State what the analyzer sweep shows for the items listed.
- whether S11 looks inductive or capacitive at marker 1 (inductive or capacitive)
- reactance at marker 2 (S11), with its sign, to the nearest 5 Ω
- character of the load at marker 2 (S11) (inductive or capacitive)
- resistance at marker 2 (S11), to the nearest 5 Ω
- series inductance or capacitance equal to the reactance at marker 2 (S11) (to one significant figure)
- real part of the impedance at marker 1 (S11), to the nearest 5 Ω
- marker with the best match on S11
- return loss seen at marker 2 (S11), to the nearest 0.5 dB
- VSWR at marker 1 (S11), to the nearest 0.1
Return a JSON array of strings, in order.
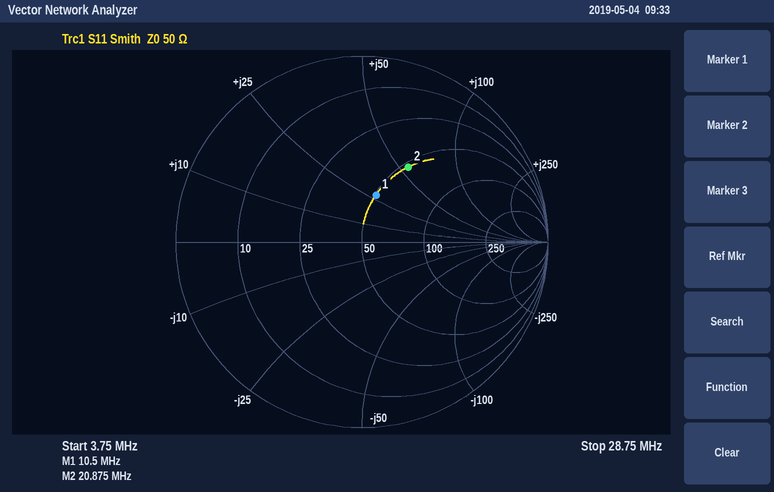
["inductive", "+55 Ω", "inductive", "55 Ω", "400 nH", "50 Ω", "marker 1", "6.5 dB", "1.7"]
